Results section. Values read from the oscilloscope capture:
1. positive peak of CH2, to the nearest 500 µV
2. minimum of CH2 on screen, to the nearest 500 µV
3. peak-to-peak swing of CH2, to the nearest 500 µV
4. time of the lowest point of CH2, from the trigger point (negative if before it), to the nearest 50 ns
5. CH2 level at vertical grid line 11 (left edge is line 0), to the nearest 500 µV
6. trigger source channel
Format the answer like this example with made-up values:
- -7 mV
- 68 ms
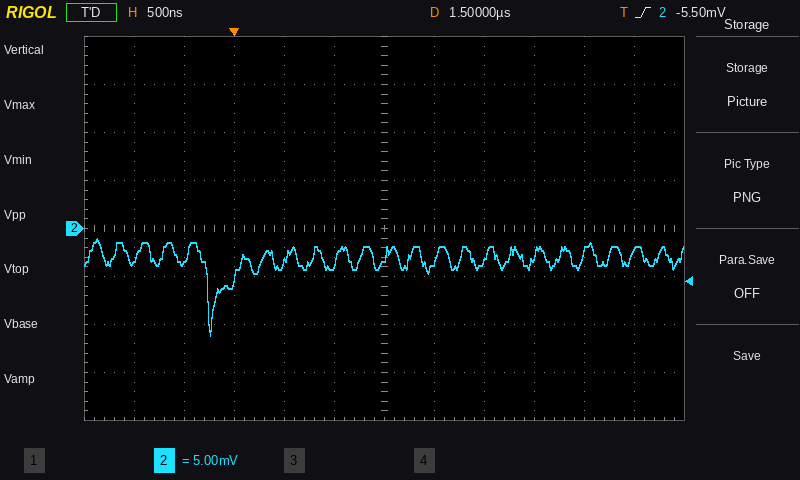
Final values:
- -1.0 mV
- -11.0 mV
- 10.0 mV
- -250 ns
- -2.5 mV
- CH2
